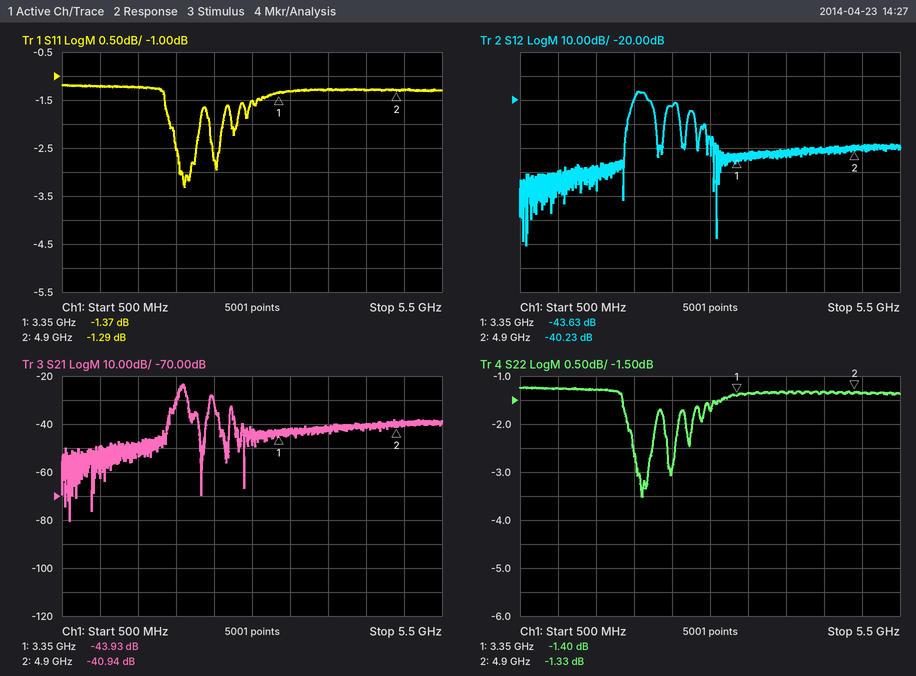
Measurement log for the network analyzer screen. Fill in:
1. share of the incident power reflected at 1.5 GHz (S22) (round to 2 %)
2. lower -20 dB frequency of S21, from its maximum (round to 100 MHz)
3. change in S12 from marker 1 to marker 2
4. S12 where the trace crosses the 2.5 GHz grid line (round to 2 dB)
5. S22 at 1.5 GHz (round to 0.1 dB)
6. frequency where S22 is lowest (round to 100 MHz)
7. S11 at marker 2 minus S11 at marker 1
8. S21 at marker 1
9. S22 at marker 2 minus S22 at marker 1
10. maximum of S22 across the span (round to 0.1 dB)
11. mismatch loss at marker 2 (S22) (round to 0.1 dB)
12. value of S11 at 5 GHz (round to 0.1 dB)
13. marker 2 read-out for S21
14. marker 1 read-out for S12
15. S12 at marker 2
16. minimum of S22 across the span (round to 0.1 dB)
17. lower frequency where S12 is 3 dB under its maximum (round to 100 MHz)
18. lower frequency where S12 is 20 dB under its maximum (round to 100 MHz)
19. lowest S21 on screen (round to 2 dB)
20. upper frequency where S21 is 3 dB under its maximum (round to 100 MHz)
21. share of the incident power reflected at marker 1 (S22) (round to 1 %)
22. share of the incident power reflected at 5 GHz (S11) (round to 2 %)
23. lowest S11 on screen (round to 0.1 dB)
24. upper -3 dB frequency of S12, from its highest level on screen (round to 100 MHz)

74 %
1.9 GHz
3.40 dB
-22 dB
-1.3 dB
2.1 GHz
0.08 dB
-43.93 dB
0.07 dB
-1.2 dB
5.8 dB
-1.3 dB
-40.94 dB
-43.63 dB
-40.23 dB
-3.5 dB
2.0 GHz
1.9 GHz
-80 dB
2.1 GHz
72 %
74 %
-3.3 dB
2.2 GHz
